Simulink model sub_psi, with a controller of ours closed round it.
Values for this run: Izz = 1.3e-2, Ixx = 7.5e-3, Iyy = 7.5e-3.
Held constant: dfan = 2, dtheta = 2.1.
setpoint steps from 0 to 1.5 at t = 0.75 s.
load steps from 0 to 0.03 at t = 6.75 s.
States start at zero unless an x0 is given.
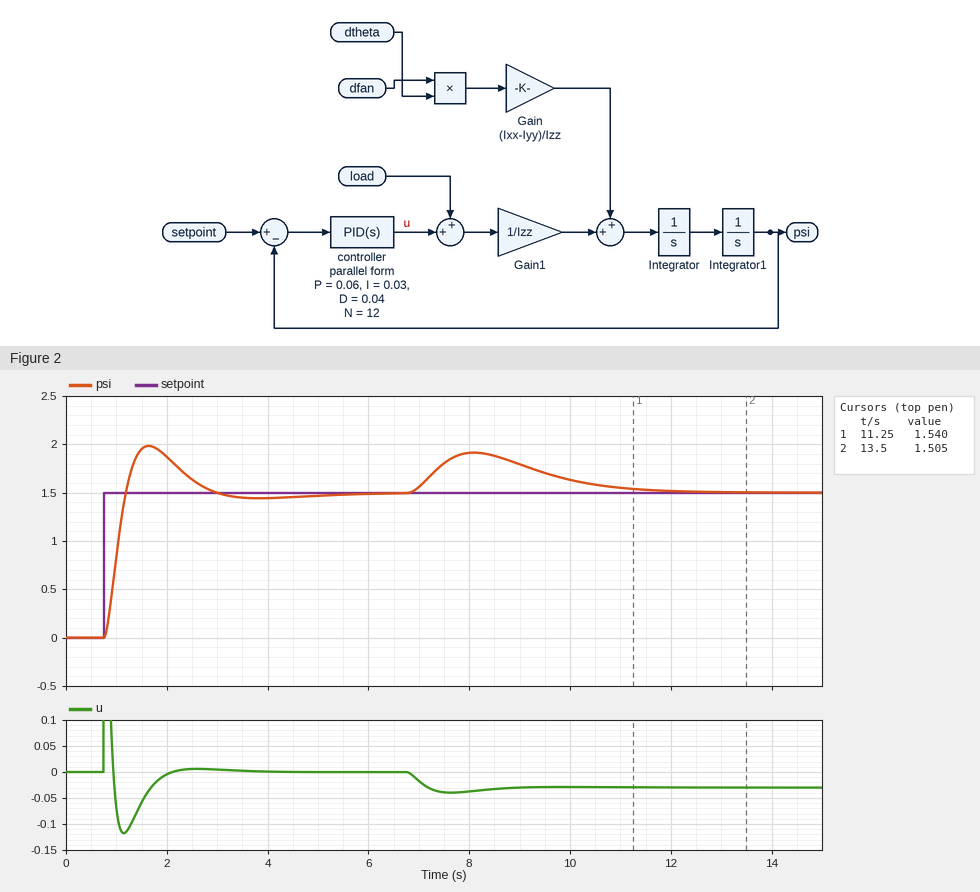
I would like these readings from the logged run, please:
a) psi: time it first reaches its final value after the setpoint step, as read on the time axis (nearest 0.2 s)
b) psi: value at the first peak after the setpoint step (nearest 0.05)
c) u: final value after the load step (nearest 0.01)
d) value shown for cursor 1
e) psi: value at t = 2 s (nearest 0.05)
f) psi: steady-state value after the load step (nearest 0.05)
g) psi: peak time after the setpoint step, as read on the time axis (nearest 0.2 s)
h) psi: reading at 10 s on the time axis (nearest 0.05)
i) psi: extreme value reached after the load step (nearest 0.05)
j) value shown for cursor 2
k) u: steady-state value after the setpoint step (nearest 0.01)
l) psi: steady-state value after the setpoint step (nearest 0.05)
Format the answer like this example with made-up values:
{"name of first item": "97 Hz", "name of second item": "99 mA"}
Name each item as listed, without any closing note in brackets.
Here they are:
{"psi: time it first reaches its final value after the setpoint step, as read on the time axis": "1.2 s", "psi: value at the first peak after the setpoint step": "2.00", "u: final value after the load step": "-0.03", "value shown for cursor 1": "1.540", "psi: value at t = 2 s": "1.85", "psi: steady-state value after the load step": "1.50", "psi: peak time after the setpoint step, as read on the time axis": "1.6 s", "psi: reading at 10 s on the time axis": "1.65", "psi: extreme value reached after the load step": "1.90", "value shown for cursor 2": "1.505", "u: steady-state value after the setpoint step": "0.00", "psi: steady-state value after the setpoint step": "1.50"}
